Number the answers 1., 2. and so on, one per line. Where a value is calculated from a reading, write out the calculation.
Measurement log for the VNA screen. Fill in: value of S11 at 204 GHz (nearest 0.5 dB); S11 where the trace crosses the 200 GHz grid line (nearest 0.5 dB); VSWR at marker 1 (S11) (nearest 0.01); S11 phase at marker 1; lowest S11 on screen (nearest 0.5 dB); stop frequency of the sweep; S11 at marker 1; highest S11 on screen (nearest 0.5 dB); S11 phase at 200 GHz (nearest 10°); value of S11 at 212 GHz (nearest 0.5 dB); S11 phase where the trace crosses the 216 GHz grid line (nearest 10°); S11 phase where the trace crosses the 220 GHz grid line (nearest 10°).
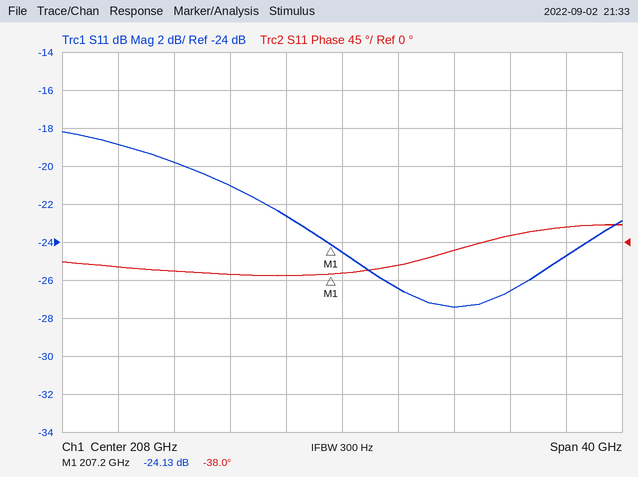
1. -22.5 dB
2. -21.0 dB
3. (1 + 0.0622)/(1 − 0.0622) ≈ 1.13
4. -38.0°
5. -27.5 dB
6. 228 GHz
7. -24.13 dB
8. -18.0 dB
9. -40°
10. -26.5 dB
11. -10°
12. 10°
